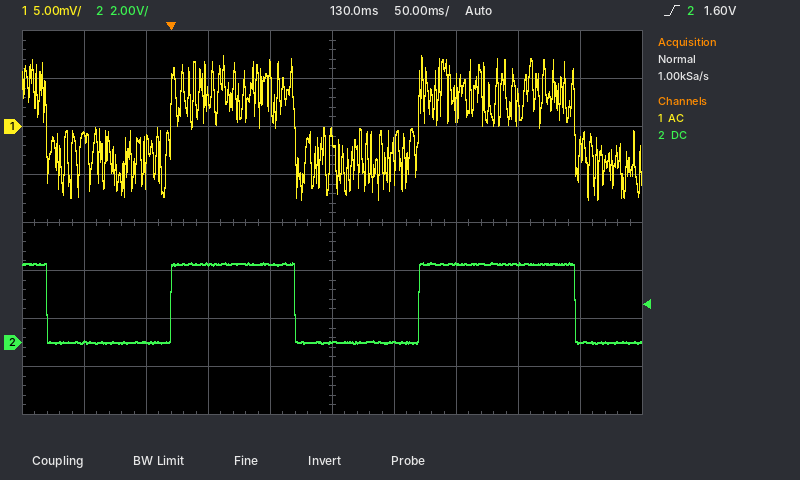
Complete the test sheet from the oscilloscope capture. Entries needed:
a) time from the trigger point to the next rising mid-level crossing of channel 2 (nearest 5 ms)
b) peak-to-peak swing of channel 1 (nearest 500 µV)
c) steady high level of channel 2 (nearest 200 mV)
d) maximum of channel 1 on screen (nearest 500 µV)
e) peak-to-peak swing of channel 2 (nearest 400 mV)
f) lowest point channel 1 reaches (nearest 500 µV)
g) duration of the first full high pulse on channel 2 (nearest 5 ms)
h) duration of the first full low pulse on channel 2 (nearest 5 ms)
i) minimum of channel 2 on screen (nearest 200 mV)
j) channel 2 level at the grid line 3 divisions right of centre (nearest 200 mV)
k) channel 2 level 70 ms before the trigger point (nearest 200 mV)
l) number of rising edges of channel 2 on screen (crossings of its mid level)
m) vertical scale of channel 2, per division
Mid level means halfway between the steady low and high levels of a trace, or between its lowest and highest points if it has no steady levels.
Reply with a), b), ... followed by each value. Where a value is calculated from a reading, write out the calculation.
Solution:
a) 200 ms
b) 7.5 mV − (-7.5 mV) = 15.0 mV
c) 3.2 V
d) 7.5 mV
e) 3.2 V
f) -7.5 mV
g) 100 ms
h) 100 ms
i) 0.0 V
j) 3.2 V
k) 0.0 V
l) 2
m) 2 V
